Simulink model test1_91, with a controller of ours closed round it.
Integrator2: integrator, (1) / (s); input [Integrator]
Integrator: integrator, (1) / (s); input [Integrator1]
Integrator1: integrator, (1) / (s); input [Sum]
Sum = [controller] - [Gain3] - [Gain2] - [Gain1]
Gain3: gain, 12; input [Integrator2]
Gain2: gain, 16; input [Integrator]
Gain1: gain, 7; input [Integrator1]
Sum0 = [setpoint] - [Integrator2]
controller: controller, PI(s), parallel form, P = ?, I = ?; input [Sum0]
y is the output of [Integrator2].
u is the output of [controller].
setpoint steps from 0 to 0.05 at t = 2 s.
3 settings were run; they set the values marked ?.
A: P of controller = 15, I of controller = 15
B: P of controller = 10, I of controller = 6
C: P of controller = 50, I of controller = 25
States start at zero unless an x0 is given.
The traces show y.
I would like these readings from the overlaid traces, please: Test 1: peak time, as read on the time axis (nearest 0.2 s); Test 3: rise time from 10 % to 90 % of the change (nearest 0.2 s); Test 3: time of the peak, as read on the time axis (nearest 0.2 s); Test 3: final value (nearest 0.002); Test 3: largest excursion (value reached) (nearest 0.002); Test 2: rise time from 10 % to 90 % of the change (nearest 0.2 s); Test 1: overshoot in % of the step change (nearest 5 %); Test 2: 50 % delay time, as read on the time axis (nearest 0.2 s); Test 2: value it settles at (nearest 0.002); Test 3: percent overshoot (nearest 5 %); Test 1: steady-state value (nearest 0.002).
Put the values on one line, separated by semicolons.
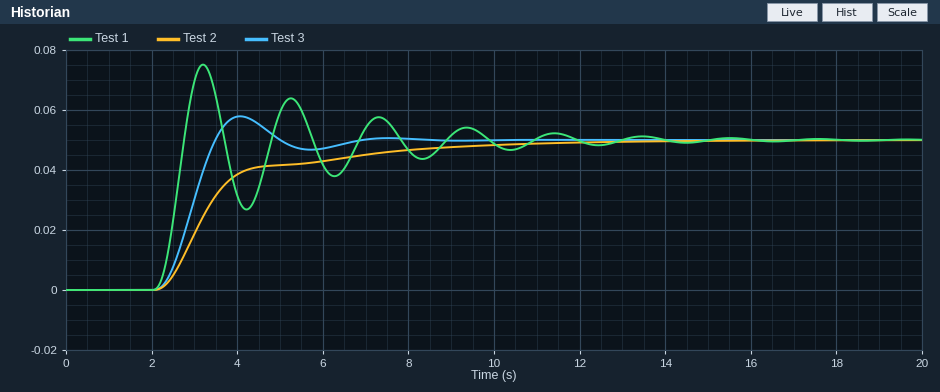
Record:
3.2 s; 1.0 s; 4.0 s; 0.050; 0.058; 4.4 s; 50 %; 3.2 s; 0.050; 15 %; 0.050
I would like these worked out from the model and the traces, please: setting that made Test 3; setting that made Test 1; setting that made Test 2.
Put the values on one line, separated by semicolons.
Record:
A; C; B
